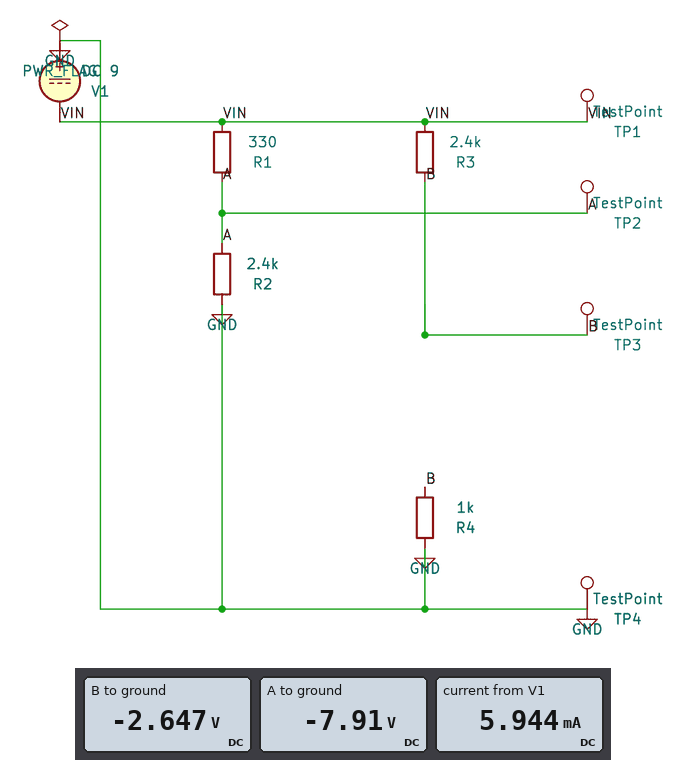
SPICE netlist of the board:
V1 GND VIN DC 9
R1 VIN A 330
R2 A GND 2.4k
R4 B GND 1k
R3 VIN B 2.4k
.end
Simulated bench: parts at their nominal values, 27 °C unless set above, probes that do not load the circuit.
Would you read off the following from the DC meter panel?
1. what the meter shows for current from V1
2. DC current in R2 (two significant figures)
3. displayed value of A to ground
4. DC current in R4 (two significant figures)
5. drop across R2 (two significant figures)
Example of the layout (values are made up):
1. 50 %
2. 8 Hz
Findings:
1. 5.944 mA
2. 3.3 mA
3. -7.91 V
4. 2.6 mA
5. 7.9 V
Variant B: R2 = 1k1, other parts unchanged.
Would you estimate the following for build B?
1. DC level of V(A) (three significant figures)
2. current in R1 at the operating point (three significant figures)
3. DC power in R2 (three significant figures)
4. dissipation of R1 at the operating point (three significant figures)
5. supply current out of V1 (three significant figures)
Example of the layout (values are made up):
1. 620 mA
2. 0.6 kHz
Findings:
1. -6.92 V
2. 6.29 mA
3. 43.6 mW
4. 13.1 mW
5. 8.94 mA
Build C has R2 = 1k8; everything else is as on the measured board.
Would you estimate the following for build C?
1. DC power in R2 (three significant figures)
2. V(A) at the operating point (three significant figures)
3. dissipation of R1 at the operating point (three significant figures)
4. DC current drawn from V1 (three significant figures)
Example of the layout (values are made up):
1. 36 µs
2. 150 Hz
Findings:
1. 32.1 mW
2. -7.61 V
3. 5.89 mW
4. 6.87 mA
